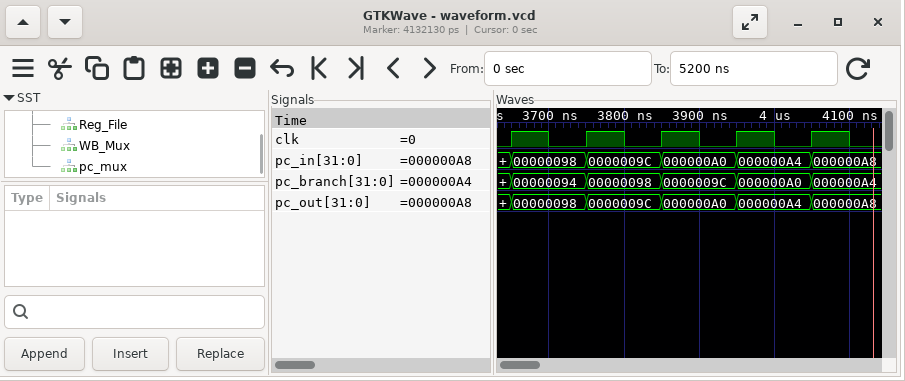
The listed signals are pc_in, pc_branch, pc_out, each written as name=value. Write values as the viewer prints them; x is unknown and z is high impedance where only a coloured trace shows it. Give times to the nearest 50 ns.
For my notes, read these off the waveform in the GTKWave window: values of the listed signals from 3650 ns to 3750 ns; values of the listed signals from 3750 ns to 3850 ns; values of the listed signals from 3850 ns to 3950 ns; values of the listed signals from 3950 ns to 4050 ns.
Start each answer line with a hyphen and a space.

- pc_in=00000098, pc_branch=00000094, pc_out=00000098
- pc_in=0000009C, pc_branch=00000098, pc_out=0000009C
- pc_in=000000A0, pc_branch=0000009C, pc_out=000000A0
- pc_in=000000A4, pc_branch=000000A0, pc_out=000000A4
